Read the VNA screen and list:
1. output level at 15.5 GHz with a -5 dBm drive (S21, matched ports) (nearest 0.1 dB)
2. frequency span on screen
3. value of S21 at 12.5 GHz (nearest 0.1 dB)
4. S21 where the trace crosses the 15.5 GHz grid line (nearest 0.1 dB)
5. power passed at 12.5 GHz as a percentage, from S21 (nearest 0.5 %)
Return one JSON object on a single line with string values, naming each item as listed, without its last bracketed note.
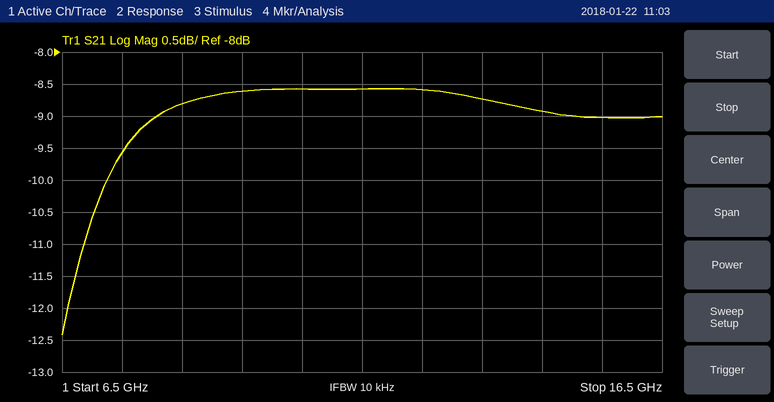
{"output level at 15.5 GHz with a -5 dBm drive (S21, matched ports)": "-14.0 dBm", "frequency span on screen": "10 GHz", "value of S21 at 12.5 GHz": "-8.6 dB", "S21 where the trace crosses the 15.5 GHz grid line": "-9.0 dB", "power passed at 12.5 GHz as a percentage, from S21": "14.0 %"}
